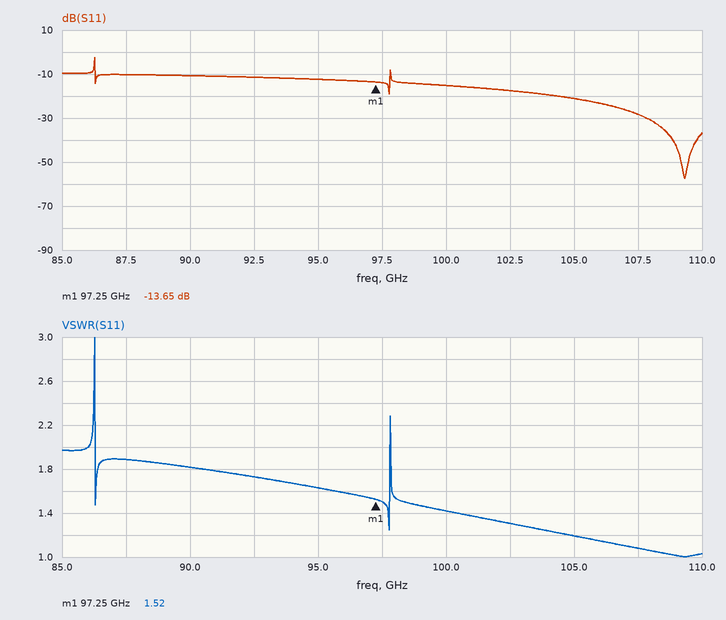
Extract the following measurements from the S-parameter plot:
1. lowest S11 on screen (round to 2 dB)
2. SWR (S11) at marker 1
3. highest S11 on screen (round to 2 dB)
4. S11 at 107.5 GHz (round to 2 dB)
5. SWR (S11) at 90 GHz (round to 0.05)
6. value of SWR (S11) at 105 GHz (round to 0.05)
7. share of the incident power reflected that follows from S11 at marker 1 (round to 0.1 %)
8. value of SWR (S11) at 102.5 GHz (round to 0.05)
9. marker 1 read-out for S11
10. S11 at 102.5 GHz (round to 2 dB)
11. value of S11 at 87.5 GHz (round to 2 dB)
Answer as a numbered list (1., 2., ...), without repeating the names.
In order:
1. -58 dB
2. 1.52
3. -2 dB
4. -28 dB
5. 1.80
6. 1.20
7. 4.3 %
8. 1.30
9. -13.65 dB
10. -18 dB
11. -10 dB
